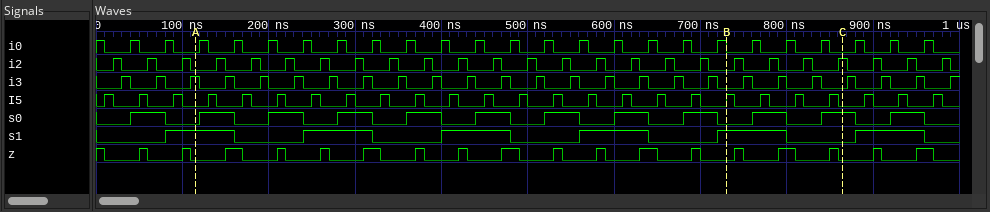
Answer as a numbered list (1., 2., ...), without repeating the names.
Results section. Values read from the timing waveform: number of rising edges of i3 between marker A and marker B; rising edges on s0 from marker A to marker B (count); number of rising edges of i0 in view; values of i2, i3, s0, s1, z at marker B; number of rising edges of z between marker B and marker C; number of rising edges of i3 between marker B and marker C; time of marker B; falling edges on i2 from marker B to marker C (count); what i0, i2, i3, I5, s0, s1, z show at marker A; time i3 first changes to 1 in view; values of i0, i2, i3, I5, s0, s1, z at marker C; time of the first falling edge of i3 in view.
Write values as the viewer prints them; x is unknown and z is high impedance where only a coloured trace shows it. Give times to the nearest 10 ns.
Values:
1. 15
2. 8
3. 24
4. i2=0, i3=0, s0=0, s1=1, z=0
5. 3
6. 3
7. 730 ns
8. 3
9. i0=0, i2=0, i3=1, I5=0, s0=0, s1=1, z=0
10. 30 ns
11. i0=0, i2=1, i3=0, I5=0, s0=1, s1=0, z=0
12. 40 ns
